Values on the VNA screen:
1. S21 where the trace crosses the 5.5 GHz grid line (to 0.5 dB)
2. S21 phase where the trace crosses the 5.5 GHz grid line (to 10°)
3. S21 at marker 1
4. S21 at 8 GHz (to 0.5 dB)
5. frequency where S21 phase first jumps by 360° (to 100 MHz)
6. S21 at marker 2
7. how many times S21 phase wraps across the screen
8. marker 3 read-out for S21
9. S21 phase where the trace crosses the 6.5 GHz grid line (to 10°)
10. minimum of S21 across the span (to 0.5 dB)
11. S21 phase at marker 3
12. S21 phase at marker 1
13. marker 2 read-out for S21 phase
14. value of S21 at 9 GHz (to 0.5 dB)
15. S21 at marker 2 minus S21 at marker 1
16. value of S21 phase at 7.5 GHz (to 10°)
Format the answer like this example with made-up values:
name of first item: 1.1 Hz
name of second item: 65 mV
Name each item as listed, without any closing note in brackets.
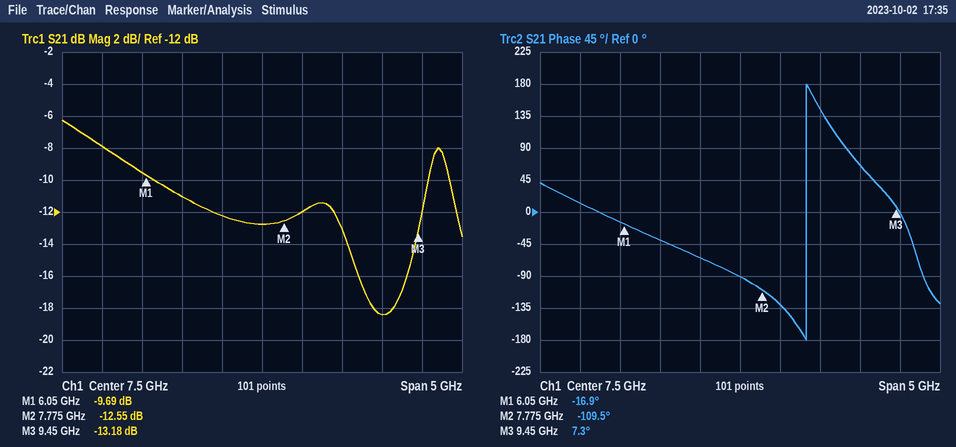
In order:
S21 where the trace crosses the 5.5 GHz grid line: -8.0 dB
S21 phase where the trace crosses the 5.5 GHz grid line: 10°
S21 at marker 1: -9.69 dB
S21 at 8 GHz: -12.0 dB
frequency where S21 phase first jumps by 360°: 8.3 GHz
S21 at marker 2: -12.55 dB
how many times S21 phase wraps across the screen: 1
marker 3 read-out for S21: -13.18 dB
S21 phase where the trace crosses the 6.5 GHz grid line: -40°
minimum of S21 across the span: -18.5 dB
S21 phase at marker 3: 7.3°
S21 phase at marker 1: -16.9°
marker 2 read-out for S21 phase: -109.5°
value of S21 at 9 GHz: -18.5 dB
S21 at marker 2 minus S21 at marker 1: -2.86 dB
value of S21 phase at 7.5 GHz: -90°
